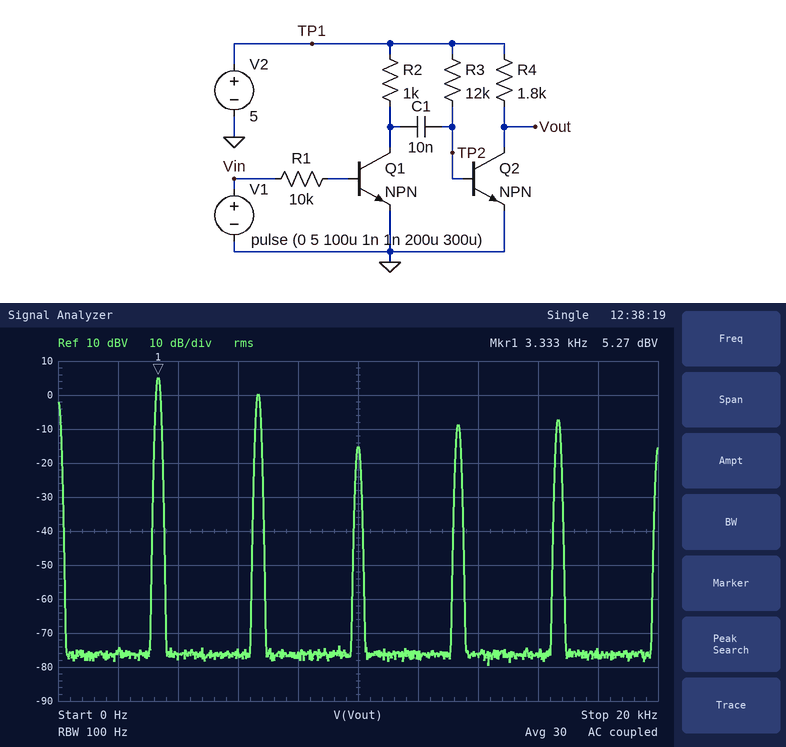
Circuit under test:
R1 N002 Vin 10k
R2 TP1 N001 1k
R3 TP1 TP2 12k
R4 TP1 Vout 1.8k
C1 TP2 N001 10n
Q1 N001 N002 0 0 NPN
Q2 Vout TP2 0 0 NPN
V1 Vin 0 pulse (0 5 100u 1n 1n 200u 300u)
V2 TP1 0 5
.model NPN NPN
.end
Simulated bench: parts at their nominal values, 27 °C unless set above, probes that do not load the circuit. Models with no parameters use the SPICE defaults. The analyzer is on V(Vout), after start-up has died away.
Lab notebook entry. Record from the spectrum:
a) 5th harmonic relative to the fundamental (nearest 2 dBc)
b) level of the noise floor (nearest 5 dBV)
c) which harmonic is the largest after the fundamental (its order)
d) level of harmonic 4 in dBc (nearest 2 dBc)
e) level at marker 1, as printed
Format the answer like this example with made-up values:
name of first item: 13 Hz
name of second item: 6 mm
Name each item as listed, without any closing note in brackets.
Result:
5th harmonic relative to the fundamental: -12 dBc
level of the noise floor: -75 dBV
which harmonic is the largest after the fundamental: 2
level of harmonic 4 in dBc: -14 dBc
level at marker 1, as printed: 5.27 dBV
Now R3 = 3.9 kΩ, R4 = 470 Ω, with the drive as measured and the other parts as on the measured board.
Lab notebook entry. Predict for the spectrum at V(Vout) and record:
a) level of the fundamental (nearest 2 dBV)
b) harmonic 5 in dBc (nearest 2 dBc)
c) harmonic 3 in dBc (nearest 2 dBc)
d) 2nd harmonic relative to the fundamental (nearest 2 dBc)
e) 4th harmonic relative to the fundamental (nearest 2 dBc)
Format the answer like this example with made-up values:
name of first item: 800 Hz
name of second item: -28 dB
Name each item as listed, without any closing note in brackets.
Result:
level of the fundamental: -4 dBV
harmonic 5 in dBc: -4 dBc
harmonic 3 in dBc: -2 dBc
2nd harmonic relative to the fundamental: 0 dBc
4th harmonic relative to the fundamental: -2 dBc
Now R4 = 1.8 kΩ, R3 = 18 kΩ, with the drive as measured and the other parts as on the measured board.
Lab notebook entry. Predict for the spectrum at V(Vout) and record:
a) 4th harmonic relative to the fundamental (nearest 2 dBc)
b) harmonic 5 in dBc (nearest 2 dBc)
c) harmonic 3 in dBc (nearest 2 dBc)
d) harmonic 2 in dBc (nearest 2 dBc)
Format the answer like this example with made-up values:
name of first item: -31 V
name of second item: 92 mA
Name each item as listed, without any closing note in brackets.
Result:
4th harmonic relative to the fundamental: -18 dBc
harmonic 5 in dBc: -16 dBc
harmonic 3 in dBc: -10 dBc
harmonic 2 in dBc: -18 dBc
